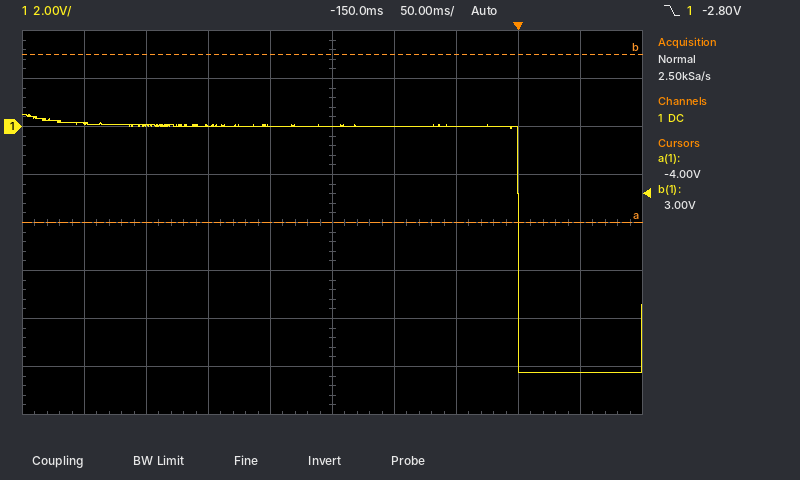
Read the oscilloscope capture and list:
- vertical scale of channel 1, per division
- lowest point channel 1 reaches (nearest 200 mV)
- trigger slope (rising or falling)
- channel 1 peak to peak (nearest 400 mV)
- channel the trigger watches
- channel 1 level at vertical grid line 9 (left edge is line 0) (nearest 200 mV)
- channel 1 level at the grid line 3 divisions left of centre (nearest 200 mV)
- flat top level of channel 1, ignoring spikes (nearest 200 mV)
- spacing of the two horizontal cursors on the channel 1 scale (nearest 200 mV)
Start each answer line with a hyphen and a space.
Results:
- 2 V
- -10.2 V
- falling
- 10.8 V
- channel 1
- -10.2 V
- 0.0 V
- 0.0 V
- 7.0 V
